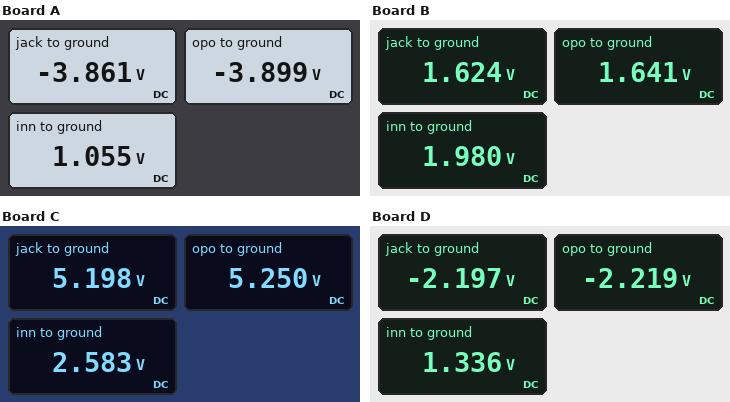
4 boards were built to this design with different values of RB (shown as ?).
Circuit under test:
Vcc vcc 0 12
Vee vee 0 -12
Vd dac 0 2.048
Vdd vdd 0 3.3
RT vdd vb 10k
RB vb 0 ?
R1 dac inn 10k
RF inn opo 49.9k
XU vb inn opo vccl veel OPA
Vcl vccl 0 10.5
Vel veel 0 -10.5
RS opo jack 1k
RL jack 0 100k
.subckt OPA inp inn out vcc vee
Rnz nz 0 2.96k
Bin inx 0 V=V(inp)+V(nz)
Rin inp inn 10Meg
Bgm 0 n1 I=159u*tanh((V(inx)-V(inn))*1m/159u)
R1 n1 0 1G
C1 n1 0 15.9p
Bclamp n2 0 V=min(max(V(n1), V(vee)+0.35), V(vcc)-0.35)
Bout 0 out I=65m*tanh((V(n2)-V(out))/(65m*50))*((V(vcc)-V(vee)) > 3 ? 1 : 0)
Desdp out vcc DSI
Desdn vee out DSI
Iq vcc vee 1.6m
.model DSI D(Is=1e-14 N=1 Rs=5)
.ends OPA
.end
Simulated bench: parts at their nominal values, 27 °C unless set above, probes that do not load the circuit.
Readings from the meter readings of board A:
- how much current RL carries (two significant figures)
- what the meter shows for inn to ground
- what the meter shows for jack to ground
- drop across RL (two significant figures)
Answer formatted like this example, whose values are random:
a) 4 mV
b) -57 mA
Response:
a) 39 µA
b) 1.055 V
c) -3.861 V
d) 3.9 V
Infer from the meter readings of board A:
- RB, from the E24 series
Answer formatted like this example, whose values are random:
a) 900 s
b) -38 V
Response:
a) 4.7 kΩ
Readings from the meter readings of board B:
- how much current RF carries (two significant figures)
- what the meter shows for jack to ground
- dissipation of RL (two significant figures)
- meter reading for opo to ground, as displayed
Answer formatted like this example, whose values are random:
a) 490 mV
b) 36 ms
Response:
a) 6.8 µA
b) 1.624 V
c) 26 µW
d) 1.641 V
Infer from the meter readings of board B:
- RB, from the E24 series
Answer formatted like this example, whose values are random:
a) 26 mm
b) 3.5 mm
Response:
a) 15 kΩ
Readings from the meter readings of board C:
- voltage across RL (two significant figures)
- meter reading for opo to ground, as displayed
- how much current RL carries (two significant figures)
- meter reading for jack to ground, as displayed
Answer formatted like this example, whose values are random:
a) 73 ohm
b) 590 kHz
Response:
a) 5.2 V
b) 5.250 V
c) 52 µA
d) 5.198 V
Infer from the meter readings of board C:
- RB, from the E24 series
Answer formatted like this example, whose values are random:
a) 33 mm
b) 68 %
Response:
a) 36 kΩ
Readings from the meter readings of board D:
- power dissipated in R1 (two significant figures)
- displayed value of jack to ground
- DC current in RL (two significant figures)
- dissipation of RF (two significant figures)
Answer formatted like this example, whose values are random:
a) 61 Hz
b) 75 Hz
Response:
a) 51 µW
b) -2.197 V
c) 22 µA
d) 250 µW
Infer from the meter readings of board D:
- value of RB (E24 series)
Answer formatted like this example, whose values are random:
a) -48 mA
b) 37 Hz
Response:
a) 6.8 kΩ
